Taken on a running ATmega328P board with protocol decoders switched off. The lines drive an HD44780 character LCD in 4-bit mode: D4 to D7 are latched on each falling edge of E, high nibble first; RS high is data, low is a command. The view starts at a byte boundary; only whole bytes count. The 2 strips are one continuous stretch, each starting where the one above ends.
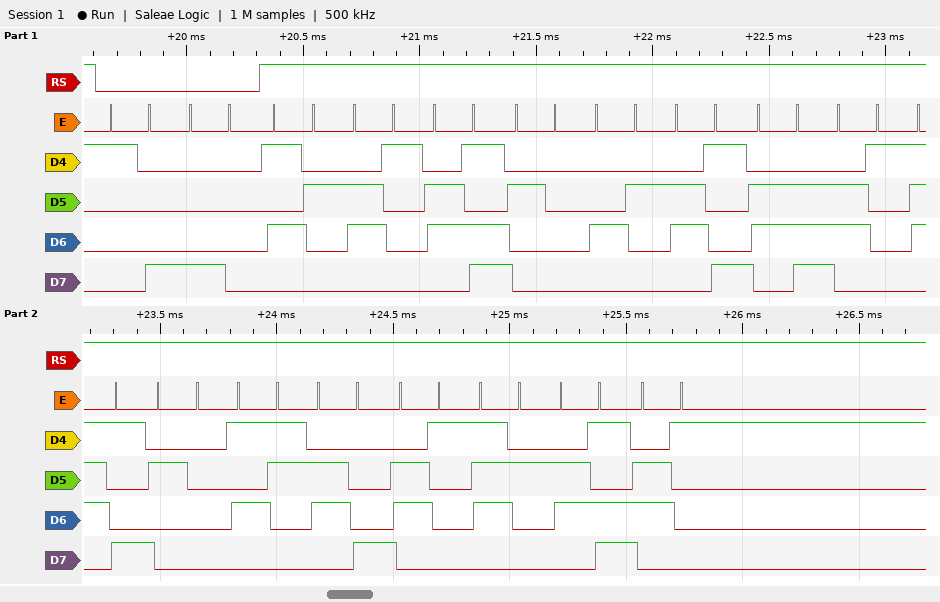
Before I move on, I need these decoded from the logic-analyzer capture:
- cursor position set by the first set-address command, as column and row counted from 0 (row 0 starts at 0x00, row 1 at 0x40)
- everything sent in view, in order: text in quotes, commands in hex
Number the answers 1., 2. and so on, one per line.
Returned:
1. column 0, row 0
2. 0x18 0x80 "Ram Binay Sharma"
